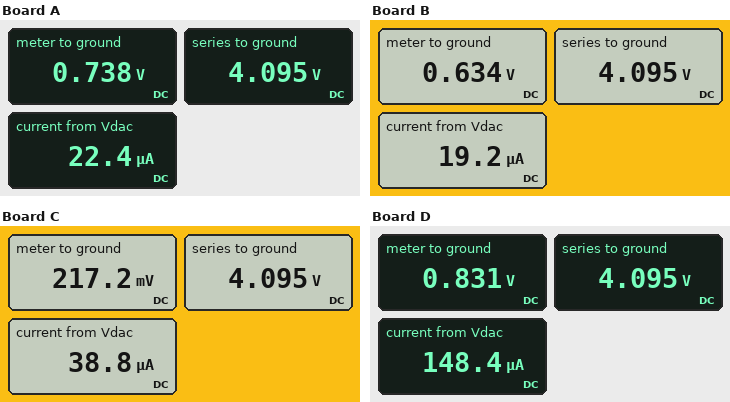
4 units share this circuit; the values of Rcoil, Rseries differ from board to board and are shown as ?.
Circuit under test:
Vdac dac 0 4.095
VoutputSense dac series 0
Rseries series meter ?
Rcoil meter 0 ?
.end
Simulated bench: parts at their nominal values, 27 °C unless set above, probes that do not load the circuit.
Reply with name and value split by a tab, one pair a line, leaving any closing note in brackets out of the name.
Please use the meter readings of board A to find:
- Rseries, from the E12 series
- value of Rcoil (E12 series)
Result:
Rseries, from the E12 series	150 kΩ
value of Rcoil	33 kΩ
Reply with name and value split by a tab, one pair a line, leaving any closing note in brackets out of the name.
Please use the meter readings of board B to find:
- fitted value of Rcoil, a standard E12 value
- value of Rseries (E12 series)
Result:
fitted value of Rcoil, a standard E12 value	33 kΩ
value of Rseries	180 kΩ
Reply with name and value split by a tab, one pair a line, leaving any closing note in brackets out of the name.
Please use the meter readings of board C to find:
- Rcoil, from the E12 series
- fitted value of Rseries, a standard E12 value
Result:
Rcoil, from the E12 series	5.6 kΩ
fitted value of Rseries, a standard E12 value	100 kΩ
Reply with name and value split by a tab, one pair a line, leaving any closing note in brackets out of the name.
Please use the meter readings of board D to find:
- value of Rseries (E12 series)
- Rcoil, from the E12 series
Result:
value of Rseries	22 kΩ
Rcoil, from the E12 series	5.6 kΩ
